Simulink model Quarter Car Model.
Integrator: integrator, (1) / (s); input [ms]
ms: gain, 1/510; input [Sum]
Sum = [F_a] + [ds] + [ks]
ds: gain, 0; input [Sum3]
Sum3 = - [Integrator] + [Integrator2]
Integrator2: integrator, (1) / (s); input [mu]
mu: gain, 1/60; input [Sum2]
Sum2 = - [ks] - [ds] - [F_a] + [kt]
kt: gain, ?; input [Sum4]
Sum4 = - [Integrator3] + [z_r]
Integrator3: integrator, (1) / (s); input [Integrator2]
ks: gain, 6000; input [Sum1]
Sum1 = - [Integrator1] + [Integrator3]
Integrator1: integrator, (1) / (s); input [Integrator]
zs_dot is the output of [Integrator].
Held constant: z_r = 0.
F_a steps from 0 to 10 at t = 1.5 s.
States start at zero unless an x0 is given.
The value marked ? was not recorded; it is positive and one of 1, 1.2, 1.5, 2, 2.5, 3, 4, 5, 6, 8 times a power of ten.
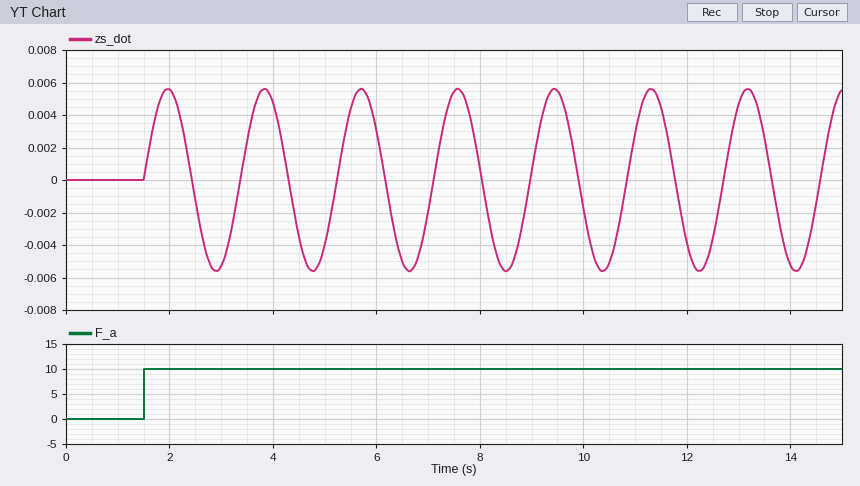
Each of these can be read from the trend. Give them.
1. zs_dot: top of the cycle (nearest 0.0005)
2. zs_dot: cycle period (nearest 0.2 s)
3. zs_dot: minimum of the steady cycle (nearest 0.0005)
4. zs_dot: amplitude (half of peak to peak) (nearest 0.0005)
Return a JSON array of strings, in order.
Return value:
["0.0055", "1.8 s", "-0.0055", "0.0055"]
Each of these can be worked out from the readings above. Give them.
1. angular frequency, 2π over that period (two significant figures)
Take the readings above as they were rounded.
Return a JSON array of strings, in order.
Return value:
["3.5 rad/s"]
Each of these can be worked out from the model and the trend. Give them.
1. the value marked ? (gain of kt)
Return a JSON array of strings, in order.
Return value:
["150000"]
